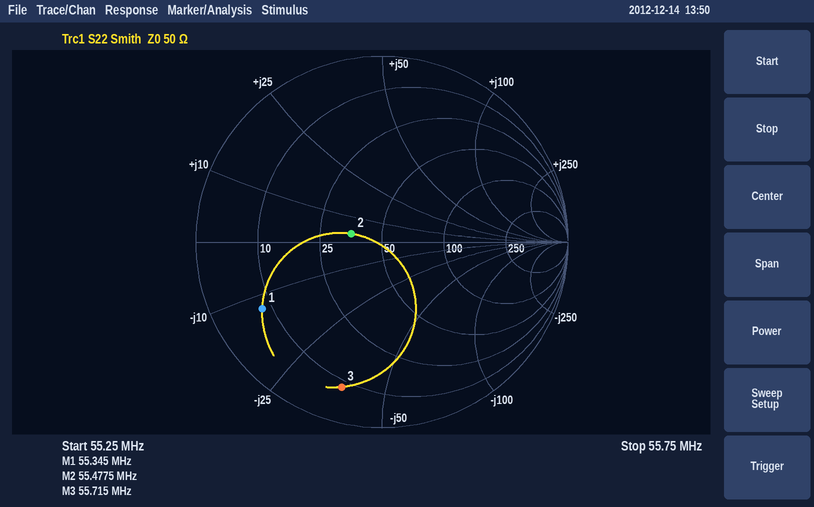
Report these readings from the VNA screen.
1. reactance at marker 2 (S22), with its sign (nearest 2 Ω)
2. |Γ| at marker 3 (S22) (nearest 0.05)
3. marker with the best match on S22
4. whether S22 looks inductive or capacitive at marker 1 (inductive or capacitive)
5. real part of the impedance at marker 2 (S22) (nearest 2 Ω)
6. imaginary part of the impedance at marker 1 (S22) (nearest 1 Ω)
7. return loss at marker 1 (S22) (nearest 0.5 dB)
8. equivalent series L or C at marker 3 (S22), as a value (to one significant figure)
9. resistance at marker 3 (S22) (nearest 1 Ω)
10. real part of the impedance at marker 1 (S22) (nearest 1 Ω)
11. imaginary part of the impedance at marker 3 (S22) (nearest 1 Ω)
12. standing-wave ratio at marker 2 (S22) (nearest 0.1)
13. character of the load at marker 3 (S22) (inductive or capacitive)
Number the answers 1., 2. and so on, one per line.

1. +4 Ω
2. 0.80
3. marker 2
4. capacitive
5. 36 Ω
6. -13 Ω
7. 2.5 dB
8. 80 pF
9. 8 Ω
10. 8 Ω
11. -37 Ω
12. 1.4
13. capacitive
